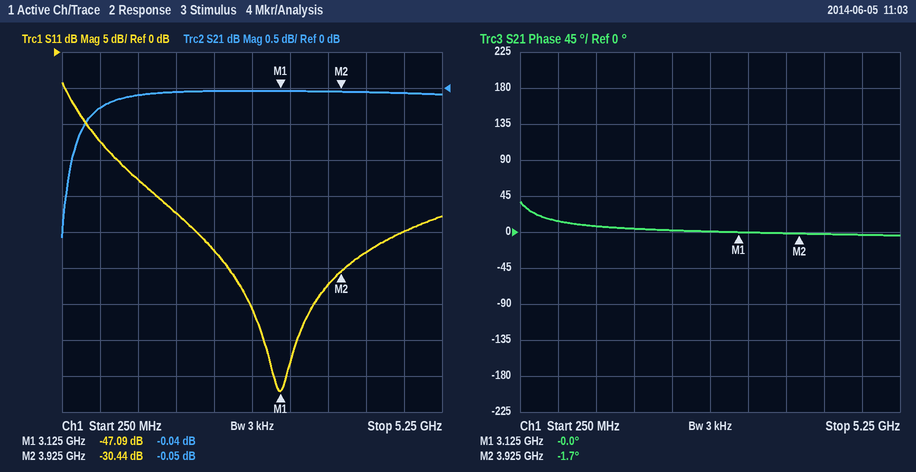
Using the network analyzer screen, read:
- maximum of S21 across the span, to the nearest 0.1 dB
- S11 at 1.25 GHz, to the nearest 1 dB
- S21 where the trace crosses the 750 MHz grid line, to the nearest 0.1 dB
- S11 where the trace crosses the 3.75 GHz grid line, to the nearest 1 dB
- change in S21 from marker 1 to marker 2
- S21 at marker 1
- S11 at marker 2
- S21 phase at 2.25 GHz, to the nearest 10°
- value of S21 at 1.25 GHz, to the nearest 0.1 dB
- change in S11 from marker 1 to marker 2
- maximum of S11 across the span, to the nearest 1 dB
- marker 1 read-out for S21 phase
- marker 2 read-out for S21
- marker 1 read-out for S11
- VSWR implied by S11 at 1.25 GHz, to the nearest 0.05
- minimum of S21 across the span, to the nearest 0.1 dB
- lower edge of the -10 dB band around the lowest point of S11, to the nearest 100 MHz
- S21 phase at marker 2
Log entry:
0.0 dB
-18 dB
-0.3 dB
-32 dB
-0.01 dB
-0.04 dB
-30.44 dB
0°
-0.1 dB
16.65 dB
-4 dB
-0.0°
-0.05 dB
-47.09 dB
1.30
-2.1 dB
600 MHz
-1.7°
